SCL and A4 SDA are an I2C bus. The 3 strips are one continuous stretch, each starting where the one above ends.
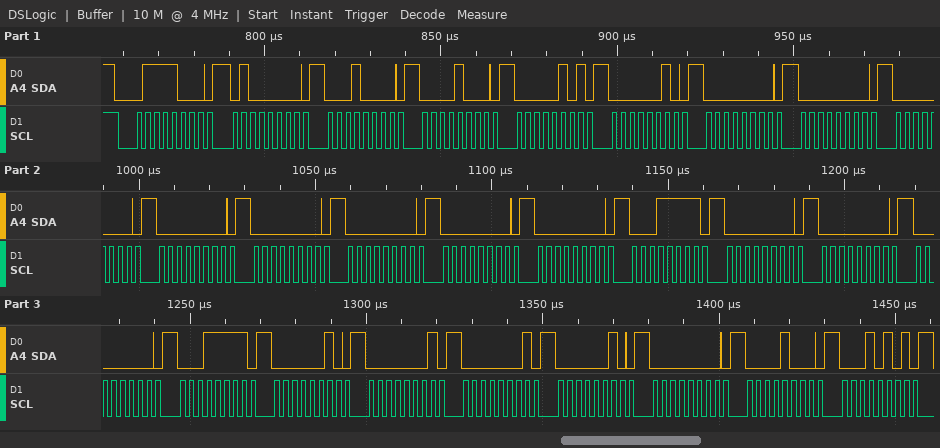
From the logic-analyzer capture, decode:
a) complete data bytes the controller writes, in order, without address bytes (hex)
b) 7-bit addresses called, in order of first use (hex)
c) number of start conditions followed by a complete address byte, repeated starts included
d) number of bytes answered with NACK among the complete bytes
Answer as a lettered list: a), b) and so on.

a) 40 10 08 05 02 00 00 00 00 00 00 00 00 1F 00 00 00 1F 02 01 01 02 00 08 15
b) 0x3C
c) 1
d) 0
